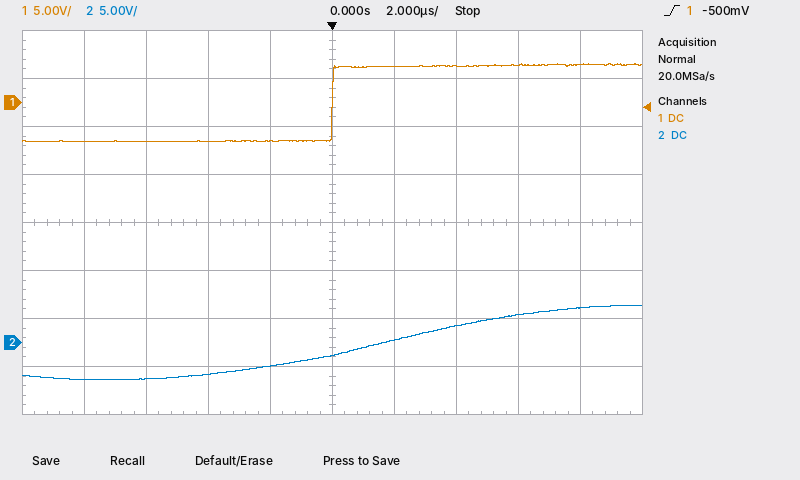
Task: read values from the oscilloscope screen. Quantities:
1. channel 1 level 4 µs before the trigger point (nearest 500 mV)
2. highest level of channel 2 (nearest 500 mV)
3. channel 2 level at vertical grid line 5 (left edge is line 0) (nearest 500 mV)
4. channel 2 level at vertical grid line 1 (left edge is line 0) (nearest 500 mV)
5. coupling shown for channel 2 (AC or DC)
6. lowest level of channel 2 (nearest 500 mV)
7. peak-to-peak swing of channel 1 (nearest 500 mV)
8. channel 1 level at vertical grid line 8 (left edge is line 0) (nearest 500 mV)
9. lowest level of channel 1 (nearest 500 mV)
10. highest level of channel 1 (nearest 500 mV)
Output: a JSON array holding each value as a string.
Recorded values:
["-4.0 V", "4.0 V", "-1.5 V", "-4.0 V", "DC", "-4.0 V", "8.0 V", "4.0 V", "-4.0 V", "4.0 V"]
